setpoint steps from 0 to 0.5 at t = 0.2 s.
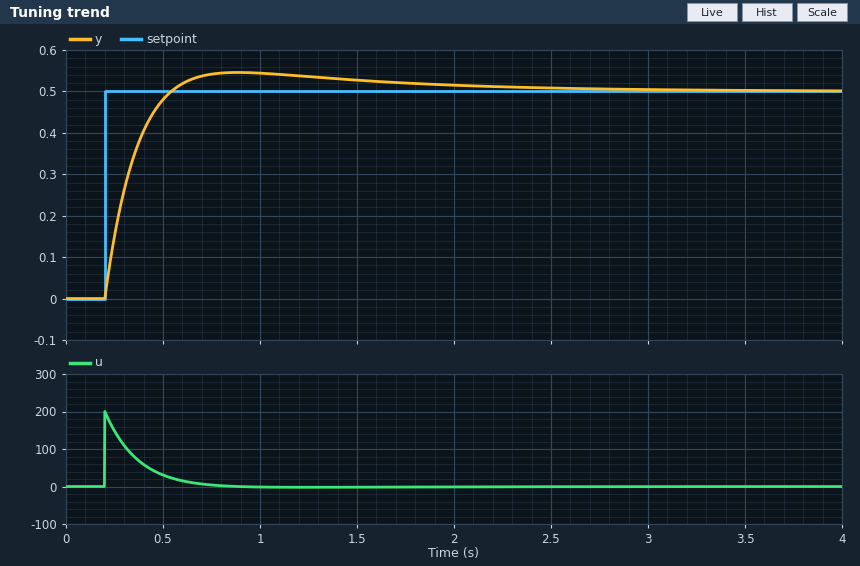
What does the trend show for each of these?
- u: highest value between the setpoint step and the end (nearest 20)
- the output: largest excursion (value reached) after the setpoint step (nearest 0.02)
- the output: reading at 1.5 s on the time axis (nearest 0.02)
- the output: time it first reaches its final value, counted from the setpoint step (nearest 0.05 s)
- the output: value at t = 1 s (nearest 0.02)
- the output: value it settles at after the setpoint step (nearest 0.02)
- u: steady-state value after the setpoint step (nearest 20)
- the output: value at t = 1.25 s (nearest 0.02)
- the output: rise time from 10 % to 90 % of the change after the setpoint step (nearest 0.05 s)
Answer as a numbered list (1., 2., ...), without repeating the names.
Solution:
1. 200
2. 0.54
3. 0.52
4. 0.35 s
5. 0.54
6. 0.50
7. 0
8. 0.54
9. 0.25 s
